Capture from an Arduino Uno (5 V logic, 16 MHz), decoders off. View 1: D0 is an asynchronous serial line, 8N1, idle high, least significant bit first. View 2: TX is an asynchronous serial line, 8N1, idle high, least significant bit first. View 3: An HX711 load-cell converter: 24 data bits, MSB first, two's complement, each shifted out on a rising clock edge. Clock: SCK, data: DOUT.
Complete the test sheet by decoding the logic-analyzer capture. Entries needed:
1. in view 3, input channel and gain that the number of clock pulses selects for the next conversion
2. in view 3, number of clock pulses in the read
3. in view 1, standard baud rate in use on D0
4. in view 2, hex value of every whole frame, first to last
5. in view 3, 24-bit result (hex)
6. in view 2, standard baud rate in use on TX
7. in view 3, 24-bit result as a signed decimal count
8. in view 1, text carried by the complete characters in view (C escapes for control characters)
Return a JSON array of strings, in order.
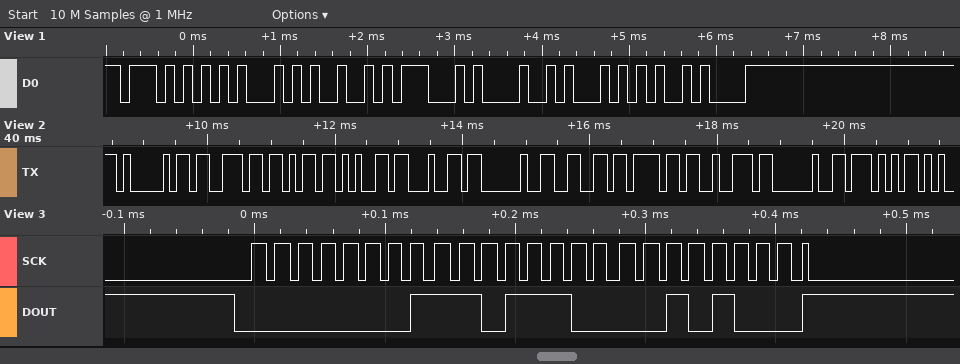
["channel A, gain 128", "25", "9600 baud", "0x41 0x73 0x6B 0x65 0x64 0x20 0x66 0x6F 0x72 0x20 0x57", "0x01DC28", "9600 baud", "121896", "\"WEIGHT\\n\""]
